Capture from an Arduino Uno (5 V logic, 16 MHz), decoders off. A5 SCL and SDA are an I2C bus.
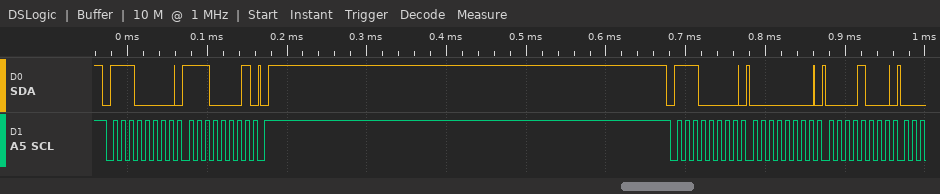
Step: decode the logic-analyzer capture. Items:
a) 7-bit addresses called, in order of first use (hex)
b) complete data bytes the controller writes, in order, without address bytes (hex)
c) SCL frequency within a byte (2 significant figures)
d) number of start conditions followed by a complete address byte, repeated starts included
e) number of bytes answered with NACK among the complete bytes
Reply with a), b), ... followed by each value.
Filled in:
a) 0x70
b) E1 00 08
c) 100 kHz
d) 2
e) 0
